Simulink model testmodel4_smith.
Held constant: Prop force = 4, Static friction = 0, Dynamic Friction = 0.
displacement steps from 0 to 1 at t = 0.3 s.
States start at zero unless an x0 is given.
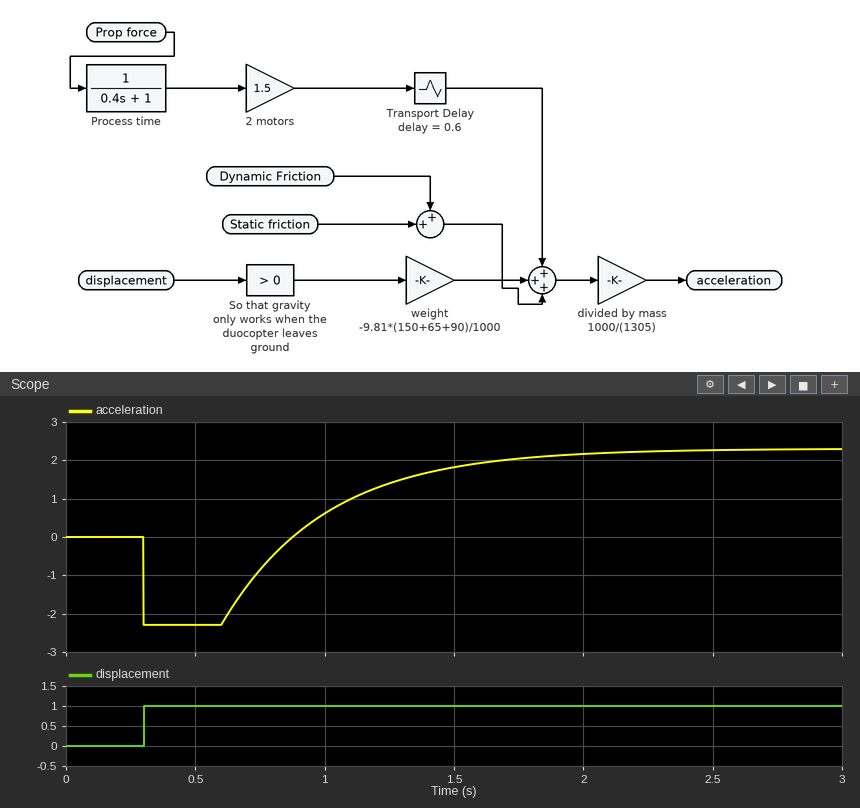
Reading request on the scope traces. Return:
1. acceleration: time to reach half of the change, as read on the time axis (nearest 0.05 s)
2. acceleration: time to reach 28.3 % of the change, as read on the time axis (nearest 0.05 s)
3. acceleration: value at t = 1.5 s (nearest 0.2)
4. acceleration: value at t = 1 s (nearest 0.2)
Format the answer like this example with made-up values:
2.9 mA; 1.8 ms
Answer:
1.15 s; 1.00 s; 1.8; 0.6
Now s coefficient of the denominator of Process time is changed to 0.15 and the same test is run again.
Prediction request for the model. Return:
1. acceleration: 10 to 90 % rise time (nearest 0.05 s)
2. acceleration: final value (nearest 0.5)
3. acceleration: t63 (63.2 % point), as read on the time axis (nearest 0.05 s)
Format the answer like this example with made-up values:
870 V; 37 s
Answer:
0.35 s; 2.5; 0.85 s
